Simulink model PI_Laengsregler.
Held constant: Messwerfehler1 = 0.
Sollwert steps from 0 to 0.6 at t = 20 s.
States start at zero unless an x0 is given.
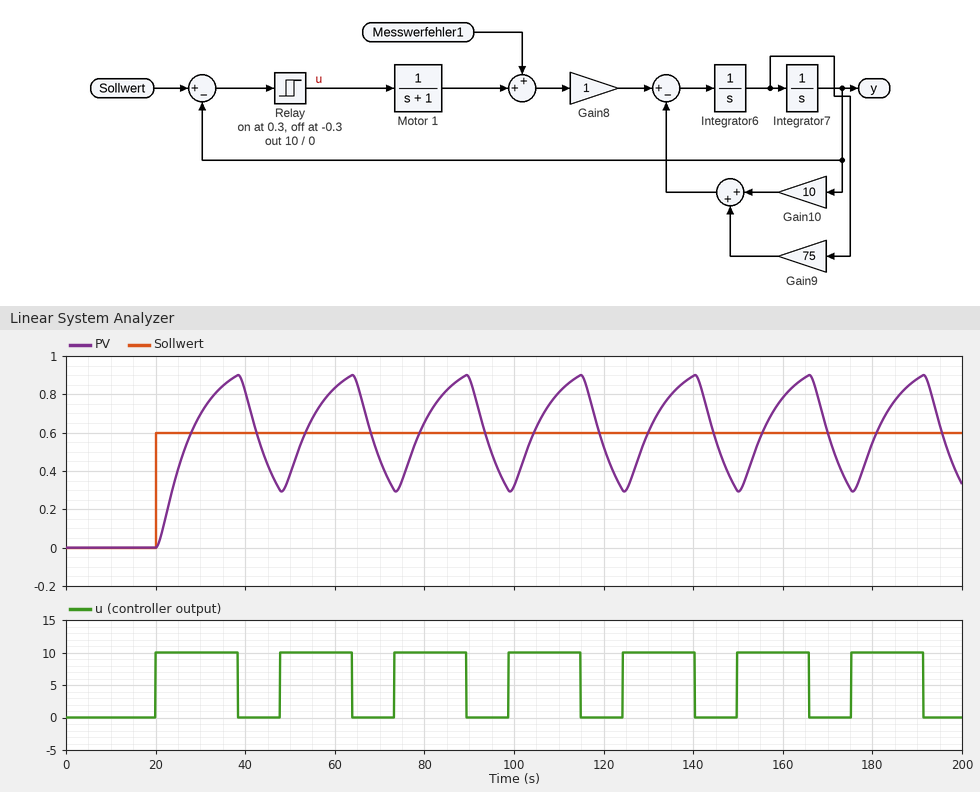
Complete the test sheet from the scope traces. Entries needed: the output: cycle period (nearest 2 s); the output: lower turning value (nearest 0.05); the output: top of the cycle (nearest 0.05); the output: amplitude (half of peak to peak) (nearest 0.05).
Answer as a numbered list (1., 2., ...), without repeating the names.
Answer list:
1. 26 s
2. 0.30
3. 0.90
4. 0.30
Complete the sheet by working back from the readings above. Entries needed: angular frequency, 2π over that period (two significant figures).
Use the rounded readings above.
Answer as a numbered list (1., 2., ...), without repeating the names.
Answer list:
1. 0.24 rad/s
